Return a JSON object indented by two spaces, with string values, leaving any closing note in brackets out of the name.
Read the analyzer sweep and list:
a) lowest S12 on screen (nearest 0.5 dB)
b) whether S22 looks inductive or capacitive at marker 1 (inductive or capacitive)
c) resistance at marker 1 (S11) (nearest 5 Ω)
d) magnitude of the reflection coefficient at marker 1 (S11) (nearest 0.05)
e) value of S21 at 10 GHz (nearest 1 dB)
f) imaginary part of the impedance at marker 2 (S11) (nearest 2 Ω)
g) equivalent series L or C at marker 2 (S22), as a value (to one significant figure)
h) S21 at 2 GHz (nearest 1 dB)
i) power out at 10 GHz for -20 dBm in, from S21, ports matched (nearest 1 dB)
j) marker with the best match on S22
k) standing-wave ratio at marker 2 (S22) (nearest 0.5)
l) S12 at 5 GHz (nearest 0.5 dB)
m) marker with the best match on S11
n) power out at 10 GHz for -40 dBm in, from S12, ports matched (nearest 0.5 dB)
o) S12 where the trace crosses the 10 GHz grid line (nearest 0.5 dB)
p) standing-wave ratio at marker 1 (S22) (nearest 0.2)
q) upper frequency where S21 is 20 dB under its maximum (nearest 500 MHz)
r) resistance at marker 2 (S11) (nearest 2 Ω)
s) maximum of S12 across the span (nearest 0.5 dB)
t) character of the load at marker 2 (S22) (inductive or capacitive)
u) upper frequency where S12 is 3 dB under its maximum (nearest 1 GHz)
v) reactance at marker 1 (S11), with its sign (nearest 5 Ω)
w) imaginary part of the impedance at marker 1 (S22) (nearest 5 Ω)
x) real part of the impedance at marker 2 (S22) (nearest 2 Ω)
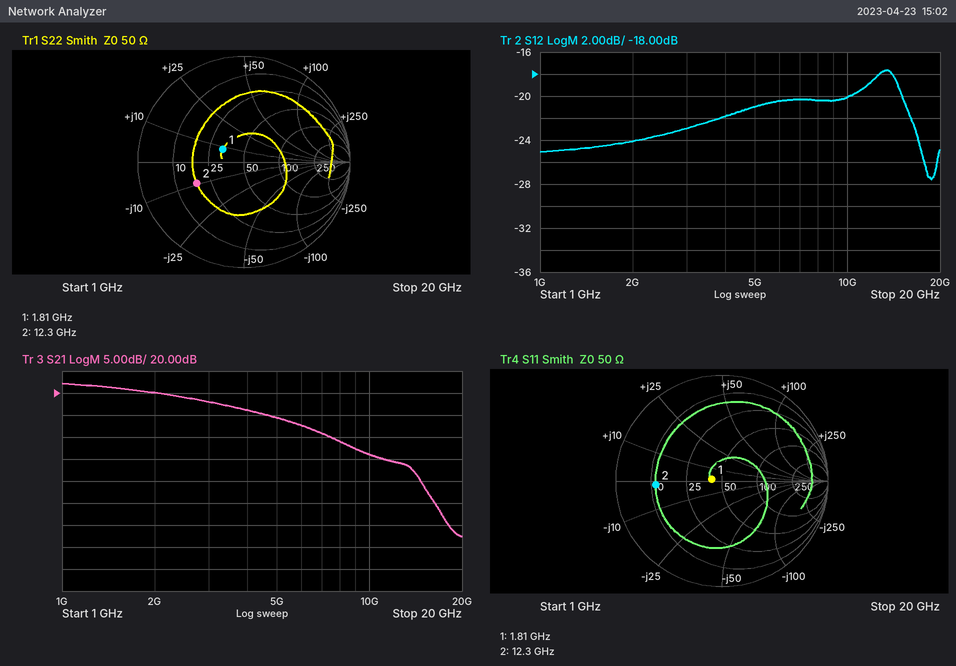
{
  "lowest S12 on screen": "-27.5 dB",
  "whether S22 looks inductive or capacitive at marker 1": "inductive",
  "resistance at marker 1 (S11)": "40 Ω",
  "magnitude of the reflection coefficient at marker 1 (S11)": "0.10",
  "value of S21 at 10 GHz": "6 dB",
  "imaginary part of the impedance at marker 2 (S11)": "-2 Ω",
  "equivalent series L or C at marker 2 (S22), as a value": "1 pF",
  "S21 at 2 GHz": "20 dB",
  "power out at 10 GHz for -20 dBm in, from S21, ports matched": "-14 dBm",
  "marker with the best match on S22": "marker 1",
  "standing-wave ratio at marker 2 (S22)": "3.0",
  "S12 at 5 GHz": "-21.0 dB",
  "marker with the best match on S11": "marker 1",
  "power out at 10 GHz for -40 dBm in, from S12, ports matched": "-60.0 dBm",
  "S12 where the trace crosses the 10 GHz grid line": "-20.0 dB",
  "standing-wave ratio at marker 1 (S22)": "1.6",
  "upper frequency where S21 is 20 dB under its maximum": "14.0 GHz",
  "resistance at marker 2 (S11)": "12 Ω",
  "maximum of S12 across the span": "-17.5 dB",
  "character of the load at marker 2 (S22)": "capacitive",
  "upper frequency where S12 is 3 dB under its maximum": "15 GHz",
  "reactance at marker 1 (S11), with its sign": "0 Ω",
  "imaginary part of the impedance at marker 1 (S22)": "+10 Ω",
  "real part of the impedance at marker 2 (S22)": "18 Ω"
}
